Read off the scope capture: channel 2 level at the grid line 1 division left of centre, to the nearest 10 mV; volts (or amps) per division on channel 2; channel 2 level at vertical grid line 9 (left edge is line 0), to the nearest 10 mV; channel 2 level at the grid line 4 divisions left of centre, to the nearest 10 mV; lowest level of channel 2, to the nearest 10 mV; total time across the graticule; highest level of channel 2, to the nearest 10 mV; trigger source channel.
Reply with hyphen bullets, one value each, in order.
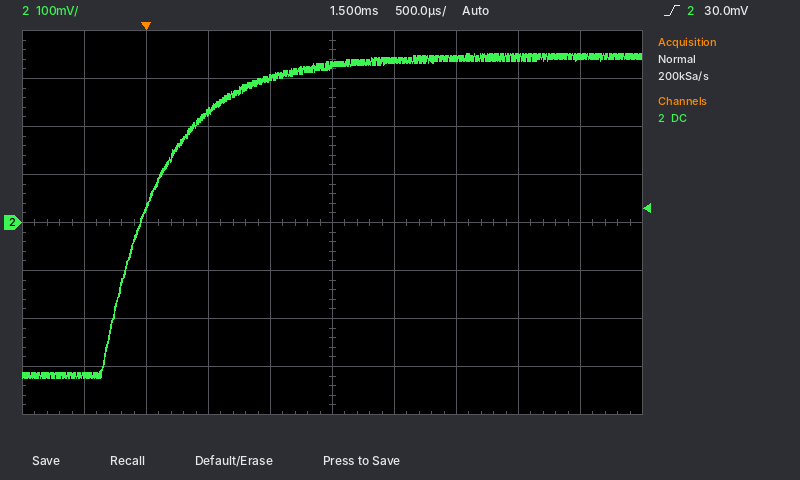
- 300 mV
- 100 mV
- 350 mV
- -320 mV
- -320 mV
- 5 ms
- 350 mV
- channel 2
